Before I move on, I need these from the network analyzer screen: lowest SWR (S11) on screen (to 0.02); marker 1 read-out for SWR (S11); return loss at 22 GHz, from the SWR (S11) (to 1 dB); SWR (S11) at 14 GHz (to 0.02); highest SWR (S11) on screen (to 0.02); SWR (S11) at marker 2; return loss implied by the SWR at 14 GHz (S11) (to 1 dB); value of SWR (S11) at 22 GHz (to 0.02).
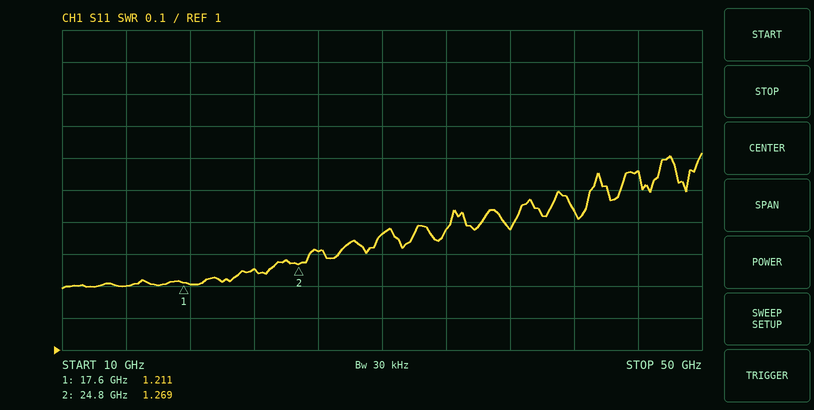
1.20
1.211
19 dB
1.20
1.62
1.269
21 dB
1.26
